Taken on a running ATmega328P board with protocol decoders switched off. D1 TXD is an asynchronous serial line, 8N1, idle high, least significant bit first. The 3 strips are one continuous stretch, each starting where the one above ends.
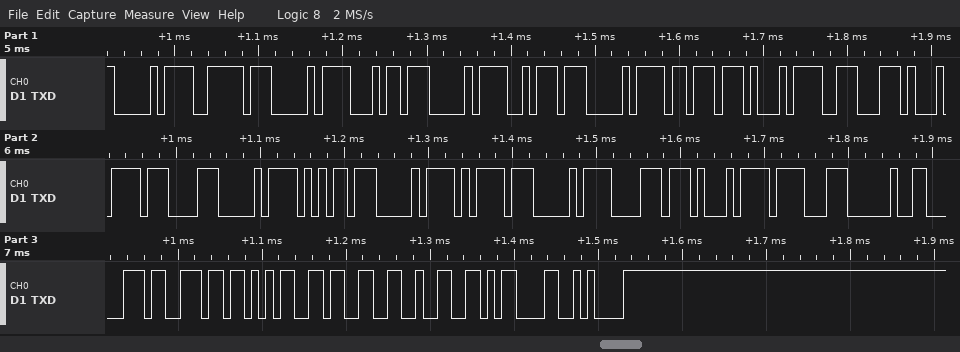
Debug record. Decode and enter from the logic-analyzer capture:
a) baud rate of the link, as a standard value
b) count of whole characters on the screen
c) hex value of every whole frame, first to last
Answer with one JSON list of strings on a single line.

["115200 baud", "28", "D0 BE D0 B4 D0 BA D0 BB D1 8E D1 87 D0 B5 D0 BD D0 B8 D1 8F 20 70 6E 35 33 32 0D 0A"]
